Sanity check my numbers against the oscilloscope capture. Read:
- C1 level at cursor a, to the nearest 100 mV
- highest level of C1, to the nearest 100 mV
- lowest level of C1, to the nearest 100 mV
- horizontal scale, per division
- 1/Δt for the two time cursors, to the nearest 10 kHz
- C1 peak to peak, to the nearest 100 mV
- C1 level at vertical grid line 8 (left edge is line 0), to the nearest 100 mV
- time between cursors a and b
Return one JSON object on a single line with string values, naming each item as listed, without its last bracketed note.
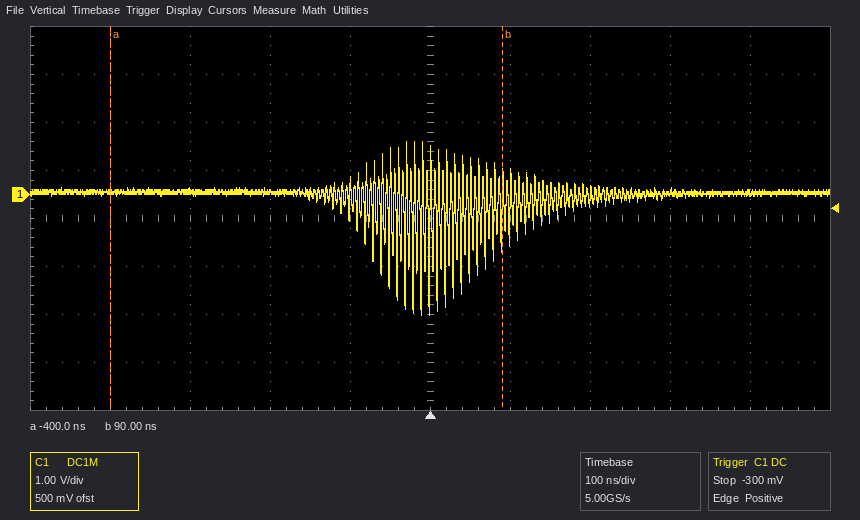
{"C1 level at cursor a, to the nearest 100 mV": "100 mV", "highest level of C1, to the nearest 100 mV": "1.1 V", "lowest level of C1, to the nearest 100 mV": "-2.5 V", "horizontal scale, per division": "100 ns", "1/Δt for the two time cursors, to the nearest 10 kHz": "2.04 MHz", "C1 peak to peak, to the nearest 100 mV": "3.6 V", "C1 level at vertical grid line 8 (left edge is line 0), to the nearest 100 mV": "100 mV", "time between cursors a and b": "490 ns"}
